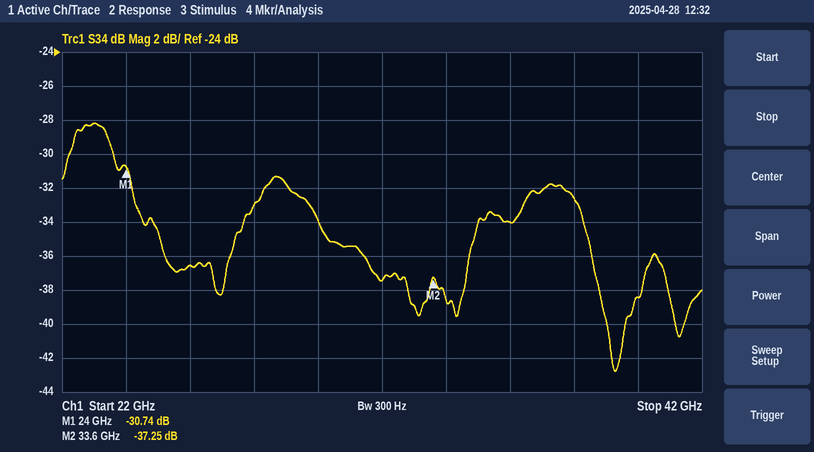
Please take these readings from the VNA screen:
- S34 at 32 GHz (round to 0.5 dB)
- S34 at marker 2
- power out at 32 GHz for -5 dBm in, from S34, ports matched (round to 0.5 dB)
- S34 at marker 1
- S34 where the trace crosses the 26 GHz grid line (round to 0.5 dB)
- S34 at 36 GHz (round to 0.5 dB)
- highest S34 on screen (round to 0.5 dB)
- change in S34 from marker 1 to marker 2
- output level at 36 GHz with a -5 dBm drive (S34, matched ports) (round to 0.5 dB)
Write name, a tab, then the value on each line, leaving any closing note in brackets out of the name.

S34 at 32 GHz	-37.5 dB
S34 at marker 2	-37.25 dB
power out at 32 GHz for -5 dBm in, from S34, ports matched	-42.5 dBm
S34 at marker 1	-30.74 dB
S34 where the trace crosses the 26 GHz grid line	-36.5 dB
S34 at 36 GHz	-34.0 dB
highest S34 on screen	-28.0 dB
change in S34 from marker 1 to marker 2	-6.51 dB
output level at 36 GHz with a -5 dBm drive (S34, matched ports)	-39.0 dBm
